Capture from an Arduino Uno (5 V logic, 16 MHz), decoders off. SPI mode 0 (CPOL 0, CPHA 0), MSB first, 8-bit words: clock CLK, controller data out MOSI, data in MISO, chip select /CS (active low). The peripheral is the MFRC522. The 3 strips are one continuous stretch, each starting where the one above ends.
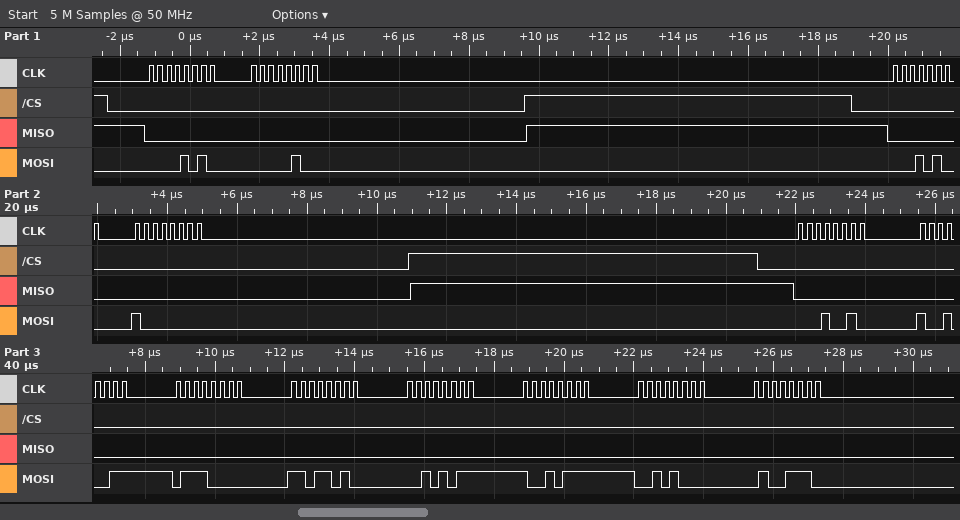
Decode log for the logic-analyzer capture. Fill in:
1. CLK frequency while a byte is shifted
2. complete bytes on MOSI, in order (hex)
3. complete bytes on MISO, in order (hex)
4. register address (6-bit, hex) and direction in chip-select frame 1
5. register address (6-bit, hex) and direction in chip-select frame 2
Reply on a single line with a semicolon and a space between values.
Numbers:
4 MHz; 0A 04 14 80 12 93 70 DA 2B 97 28 4E; 00 00 00 00 00 00 00 00 00 00 00 00; 0x05 write; 0x0A write
